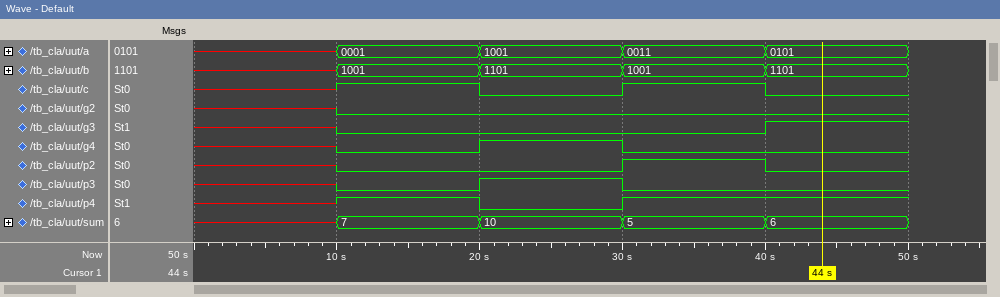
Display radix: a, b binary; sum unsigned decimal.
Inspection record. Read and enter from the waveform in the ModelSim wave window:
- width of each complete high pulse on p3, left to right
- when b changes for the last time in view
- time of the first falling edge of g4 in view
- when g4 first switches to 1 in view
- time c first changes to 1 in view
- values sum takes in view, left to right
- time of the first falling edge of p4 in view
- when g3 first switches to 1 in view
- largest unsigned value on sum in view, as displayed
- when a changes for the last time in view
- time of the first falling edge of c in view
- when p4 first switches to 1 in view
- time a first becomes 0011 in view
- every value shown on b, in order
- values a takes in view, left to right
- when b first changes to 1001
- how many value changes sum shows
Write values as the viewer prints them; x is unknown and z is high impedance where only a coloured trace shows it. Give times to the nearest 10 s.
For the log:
10 s
40 s
30 s
20 s
10 s
x, 7, 10, 5, 6
20 s
40 s
10
40 s
20 s
10 s
30 s
x, 1001, 1101, 1001, 1101
x, 0001, 1001, 0011, 0101
10 s
4
